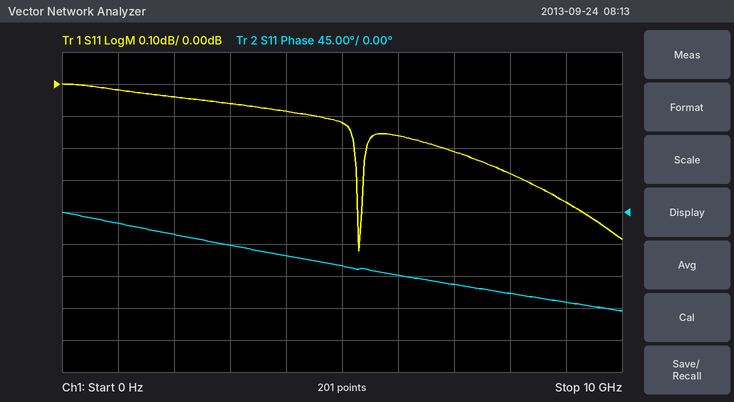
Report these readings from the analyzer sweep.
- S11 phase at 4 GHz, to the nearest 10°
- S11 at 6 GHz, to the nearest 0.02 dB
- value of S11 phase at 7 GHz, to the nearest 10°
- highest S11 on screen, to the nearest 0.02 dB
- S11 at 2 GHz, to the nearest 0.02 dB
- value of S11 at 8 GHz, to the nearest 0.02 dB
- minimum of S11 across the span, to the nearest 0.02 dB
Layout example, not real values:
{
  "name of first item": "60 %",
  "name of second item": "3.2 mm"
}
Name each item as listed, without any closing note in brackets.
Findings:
{
  "S11 phase at 4 GHz, to the nearest 10°": "-60°",
  "S11 at 6 GHz, to the nearest 0.02 dB": "-0.16 dB",
  "value of S11 phase at 7 GHz, to the nearest 10°": "-100°",
  "highest S11 on screen, to the nearest 0.02 dB": "0.00 dB",
  "S11 at 2 GHz, to the nearest 0.02 dB": "-0.04 dB",
  "value of S11 at 8 GHz, to the nearest 0.02 dB": "-0.28 dB",
  "minimum of S11 across the span, to the nearest 0.02 dB": "-0.52 dB"
}
